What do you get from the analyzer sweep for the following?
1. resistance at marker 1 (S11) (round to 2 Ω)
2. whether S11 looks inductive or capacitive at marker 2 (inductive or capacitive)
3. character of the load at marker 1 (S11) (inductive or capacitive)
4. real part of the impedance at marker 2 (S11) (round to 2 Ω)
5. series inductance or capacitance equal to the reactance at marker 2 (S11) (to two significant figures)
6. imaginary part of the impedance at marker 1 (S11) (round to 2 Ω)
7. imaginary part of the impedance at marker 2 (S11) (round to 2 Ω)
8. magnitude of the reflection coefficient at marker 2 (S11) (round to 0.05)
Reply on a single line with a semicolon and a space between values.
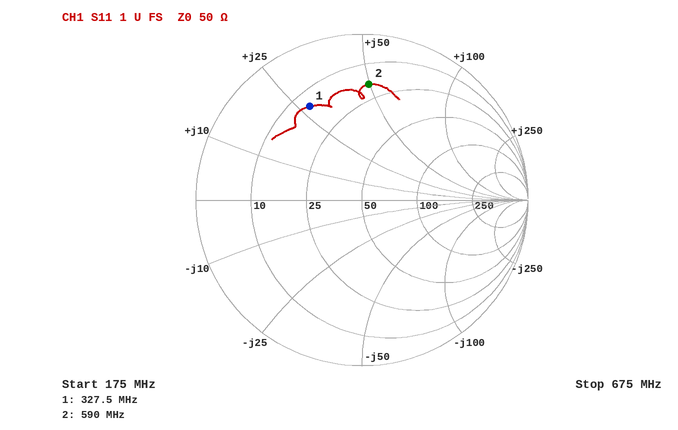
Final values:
14 Ω; inductive; inductive; 18 Ω; 13 nH; +28 Ω; +50 Ω; 0.70
